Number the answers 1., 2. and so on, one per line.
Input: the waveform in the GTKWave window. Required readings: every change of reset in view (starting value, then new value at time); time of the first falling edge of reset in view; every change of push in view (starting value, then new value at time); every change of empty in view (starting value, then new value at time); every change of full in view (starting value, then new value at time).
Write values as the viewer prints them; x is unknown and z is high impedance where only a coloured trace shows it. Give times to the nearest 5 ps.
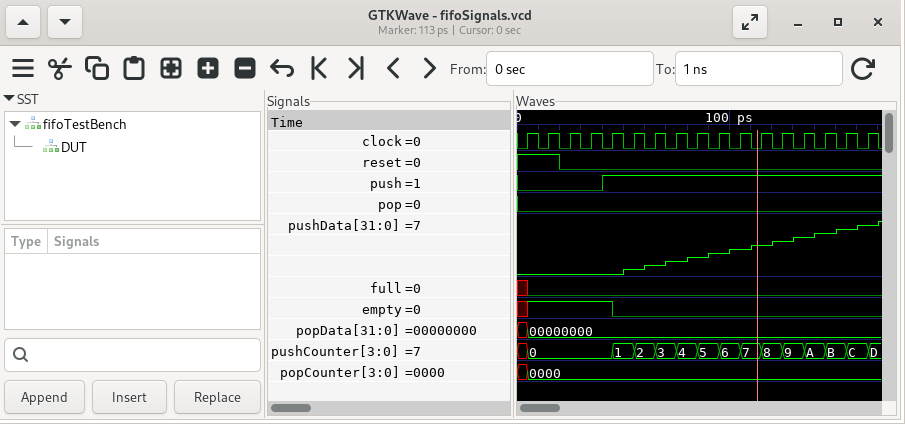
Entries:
1. 1, 0 at 20 ps
2. 20 ps
3. 0, 1 at 40 ps
4. x, 1 at 5 ps, 0 at 45 ps
5. x, 0 at 5 ps
